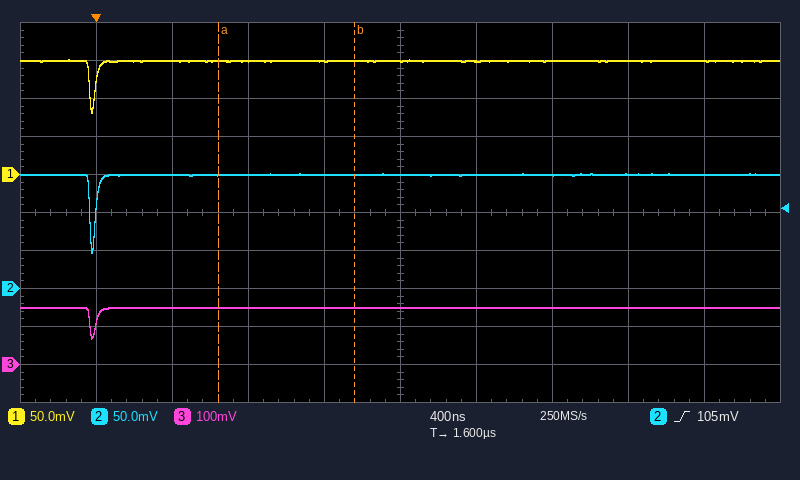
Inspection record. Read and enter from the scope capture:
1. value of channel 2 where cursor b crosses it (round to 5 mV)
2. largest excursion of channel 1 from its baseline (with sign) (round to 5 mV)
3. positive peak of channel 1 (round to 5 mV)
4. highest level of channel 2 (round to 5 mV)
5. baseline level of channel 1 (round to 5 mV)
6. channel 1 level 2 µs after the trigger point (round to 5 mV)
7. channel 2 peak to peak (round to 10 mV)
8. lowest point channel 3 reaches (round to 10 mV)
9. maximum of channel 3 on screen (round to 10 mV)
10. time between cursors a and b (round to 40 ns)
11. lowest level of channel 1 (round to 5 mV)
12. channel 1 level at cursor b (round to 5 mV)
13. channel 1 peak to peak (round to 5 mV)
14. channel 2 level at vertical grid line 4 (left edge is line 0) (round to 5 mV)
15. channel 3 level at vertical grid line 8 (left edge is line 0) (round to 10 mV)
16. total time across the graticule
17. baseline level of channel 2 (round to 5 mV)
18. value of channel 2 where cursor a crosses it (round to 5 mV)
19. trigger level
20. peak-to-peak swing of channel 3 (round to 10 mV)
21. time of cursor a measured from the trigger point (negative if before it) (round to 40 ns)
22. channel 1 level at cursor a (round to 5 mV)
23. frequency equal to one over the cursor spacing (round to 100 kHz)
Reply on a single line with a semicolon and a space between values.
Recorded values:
150 mV; -70 mV; 150 mV; 150 mV; 150 mV; 150 mV; 100 mV; 70 mV; 150 mV; 720 ns; 80 mV; 150 mV; 70 mV; 150 mV; 150 mV; 4 µs; 150 mV; 150 mV; 105 mV; 80 mV; +640 ns; 150 mV; 1.4 MHz
